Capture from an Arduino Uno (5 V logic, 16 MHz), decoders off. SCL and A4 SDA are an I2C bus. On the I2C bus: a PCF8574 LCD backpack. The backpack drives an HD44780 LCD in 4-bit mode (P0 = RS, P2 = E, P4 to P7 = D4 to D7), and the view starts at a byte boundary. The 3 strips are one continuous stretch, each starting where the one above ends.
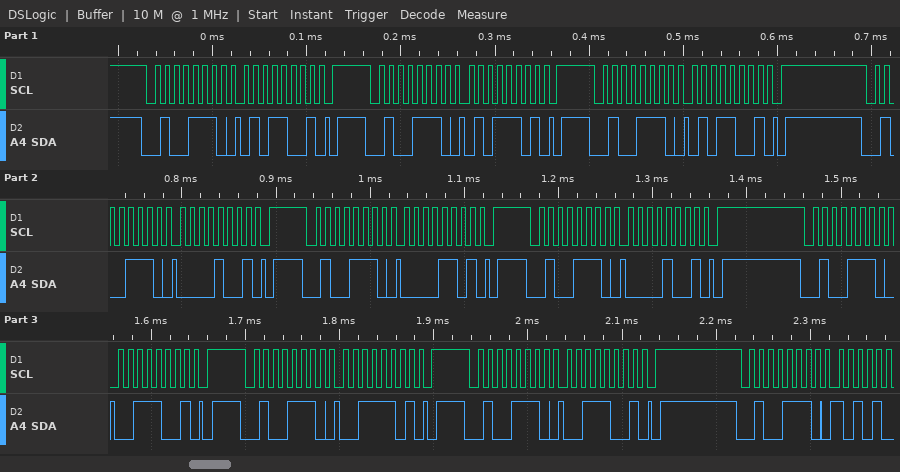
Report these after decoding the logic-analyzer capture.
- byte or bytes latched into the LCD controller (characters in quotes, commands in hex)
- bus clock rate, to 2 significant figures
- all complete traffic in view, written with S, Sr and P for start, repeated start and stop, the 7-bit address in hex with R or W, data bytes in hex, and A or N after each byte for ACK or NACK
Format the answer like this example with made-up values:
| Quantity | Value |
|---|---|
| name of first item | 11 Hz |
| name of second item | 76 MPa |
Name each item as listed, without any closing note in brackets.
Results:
| Quantity | Value |
|---|---|
| byte or bytes latched into the LCD controller | 'P' |
| bus clock rate, to 2 significant figures | 100 kHz |
| all complete traffic in view, written with S, Sr and P for start, repeated start and stop, the 7-bit address in hex with R or W, data bytes in hex, and A or N after each byte for ACK or NACK | S 27W A 59 A P S 27W A 5D A P S 27W A 59 A P S 27W A 09 A P S 27W A 0D A P S 27W A 09 A P S 27W A 39 A P S 27W A 3D A P S 27W A 39 A P S 27W A |
